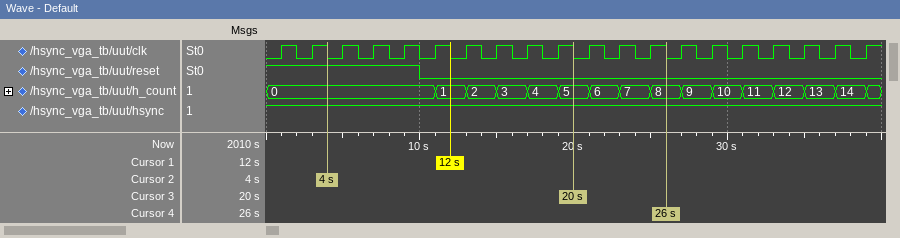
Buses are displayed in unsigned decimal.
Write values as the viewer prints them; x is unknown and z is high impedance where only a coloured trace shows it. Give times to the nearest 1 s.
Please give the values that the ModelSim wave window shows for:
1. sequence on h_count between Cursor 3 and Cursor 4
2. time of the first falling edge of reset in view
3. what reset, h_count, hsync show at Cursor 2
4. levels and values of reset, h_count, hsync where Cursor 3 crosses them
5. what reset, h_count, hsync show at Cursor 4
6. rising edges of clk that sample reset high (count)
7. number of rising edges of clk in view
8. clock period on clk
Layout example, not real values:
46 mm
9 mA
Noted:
5, 6, 7, 8
10 s
reset=1, h_count=0, hsync=1
reset=0, h_count=5, hsync=1
reset=0, h_count=8, hsync=1
5
20
2 s
